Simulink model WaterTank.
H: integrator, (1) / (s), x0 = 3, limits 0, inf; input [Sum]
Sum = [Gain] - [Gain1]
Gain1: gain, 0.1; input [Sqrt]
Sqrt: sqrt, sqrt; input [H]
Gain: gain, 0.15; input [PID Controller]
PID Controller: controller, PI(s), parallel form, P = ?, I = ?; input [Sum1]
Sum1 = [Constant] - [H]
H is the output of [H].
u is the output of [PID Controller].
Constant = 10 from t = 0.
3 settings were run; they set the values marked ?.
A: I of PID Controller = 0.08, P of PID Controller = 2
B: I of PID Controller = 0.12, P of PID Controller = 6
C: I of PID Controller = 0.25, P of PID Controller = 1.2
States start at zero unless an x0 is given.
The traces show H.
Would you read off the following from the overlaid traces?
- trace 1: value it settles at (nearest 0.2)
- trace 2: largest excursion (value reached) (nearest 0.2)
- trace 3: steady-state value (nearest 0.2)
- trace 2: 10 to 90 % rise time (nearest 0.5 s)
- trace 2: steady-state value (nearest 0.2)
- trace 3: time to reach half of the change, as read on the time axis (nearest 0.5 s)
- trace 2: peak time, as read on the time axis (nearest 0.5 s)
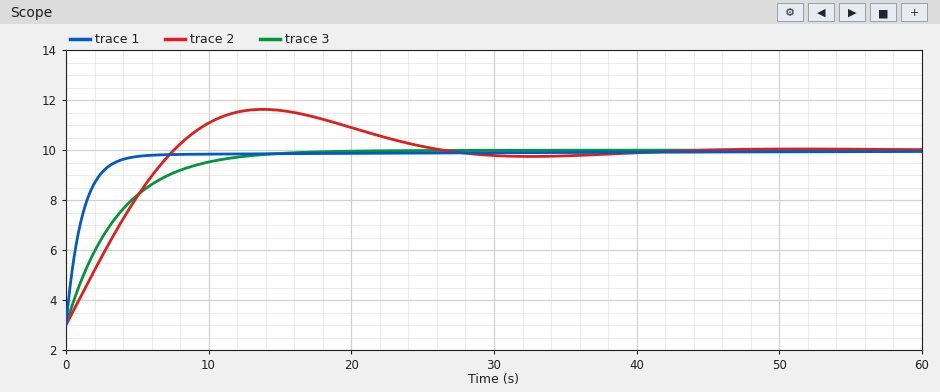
10.0
11.6
10.0
6.0 s
10.0
2.5 s
14.0 s
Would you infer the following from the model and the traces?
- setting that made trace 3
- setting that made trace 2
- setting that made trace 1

A
C
B
